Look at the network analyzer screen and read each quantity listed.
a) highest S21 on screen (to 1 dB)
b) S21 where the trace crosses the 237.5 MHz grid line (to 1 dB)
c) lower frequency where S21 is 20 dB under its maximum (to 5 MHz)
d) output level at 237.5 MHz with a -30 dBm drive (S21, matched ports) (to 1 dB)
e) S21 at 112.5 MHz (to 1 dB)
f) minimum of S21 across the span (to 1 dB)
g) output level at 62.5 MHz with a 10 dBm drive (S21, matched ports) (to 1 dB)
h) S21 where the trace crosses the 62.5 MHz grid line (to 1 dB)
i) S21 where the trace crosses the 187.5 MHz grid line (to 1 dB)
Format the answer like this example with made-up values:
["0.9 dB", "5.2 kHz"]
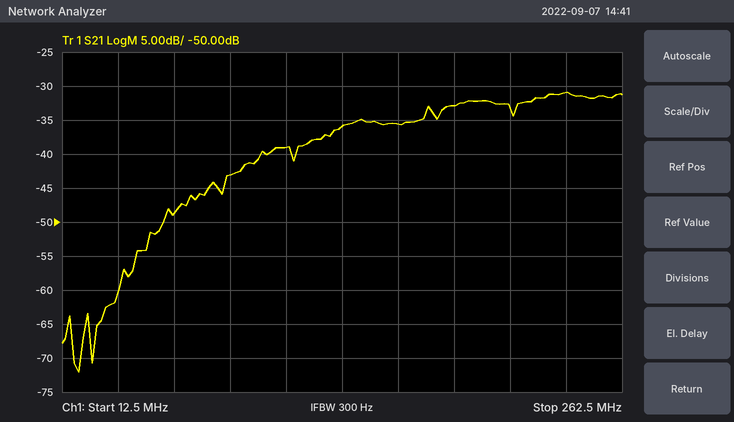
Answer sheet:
["-31 dB", "-31 dB", "55 MHz", "-61 dBm", "-39 dB", "-72 dB", "-39 dBm", "-49 dB", "-33 dB"]
